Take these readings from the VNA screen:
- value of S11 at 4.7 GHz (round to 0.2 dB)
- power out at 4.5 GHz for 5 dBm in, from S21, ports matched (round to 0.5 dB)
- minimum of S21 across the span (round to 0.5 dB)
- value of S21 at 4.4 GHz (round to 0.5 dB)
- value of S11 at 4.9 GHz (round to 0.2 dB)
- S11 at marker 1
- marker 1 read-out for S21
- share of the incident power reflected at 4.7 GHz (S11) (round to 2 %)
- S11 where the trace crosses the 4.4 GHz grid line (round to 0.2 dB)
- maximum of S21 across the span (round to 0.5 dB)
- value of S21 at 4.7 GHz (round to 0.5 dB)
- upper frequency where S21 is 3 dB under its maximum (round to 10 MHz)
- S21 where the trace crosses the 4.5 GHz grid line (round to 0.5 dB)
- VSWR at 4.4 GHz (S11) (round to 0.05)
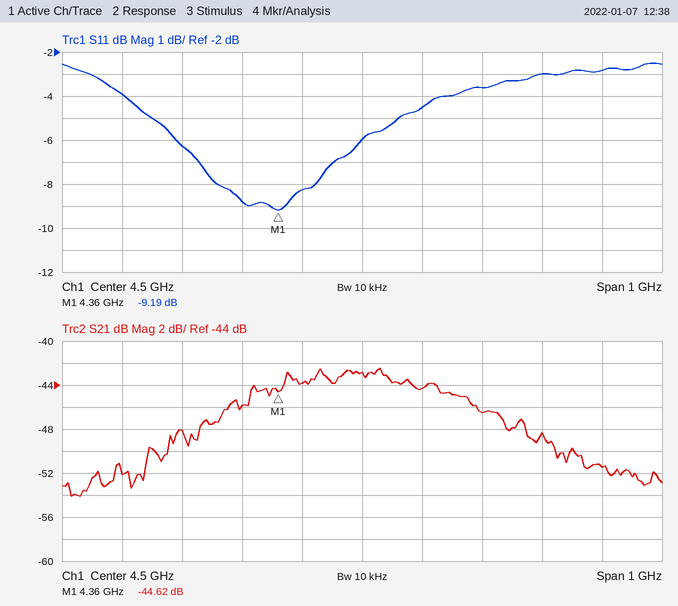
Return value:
-3.6 dB
-38.0 dBm
-54.0 dB
-44.0 dB
-2.8 dB
-9.19 dB
-44.62 dB
44 %
-8.2 dB
-42.5 dB
-46.5 dB
4.68 GHz
-43.0 dB
2.25
